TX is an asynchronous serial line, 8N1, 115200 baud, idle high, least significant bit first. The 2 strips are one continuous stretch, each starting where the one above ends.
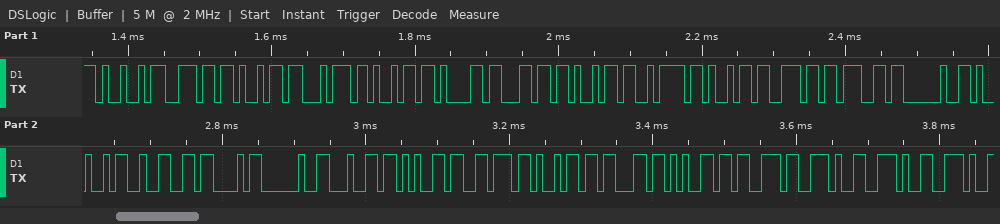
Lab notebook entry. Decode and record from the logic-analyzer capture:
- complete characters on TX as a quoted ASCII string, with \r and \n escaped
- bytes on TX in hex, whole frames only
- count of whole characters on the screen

"Initializing I2C devices..."
49 6E 69 74 69 61 6C 69 7A 69 6E 67 20 49 32 43 20 64 65 76 69 63 65 73 2E 2E 2E
27
